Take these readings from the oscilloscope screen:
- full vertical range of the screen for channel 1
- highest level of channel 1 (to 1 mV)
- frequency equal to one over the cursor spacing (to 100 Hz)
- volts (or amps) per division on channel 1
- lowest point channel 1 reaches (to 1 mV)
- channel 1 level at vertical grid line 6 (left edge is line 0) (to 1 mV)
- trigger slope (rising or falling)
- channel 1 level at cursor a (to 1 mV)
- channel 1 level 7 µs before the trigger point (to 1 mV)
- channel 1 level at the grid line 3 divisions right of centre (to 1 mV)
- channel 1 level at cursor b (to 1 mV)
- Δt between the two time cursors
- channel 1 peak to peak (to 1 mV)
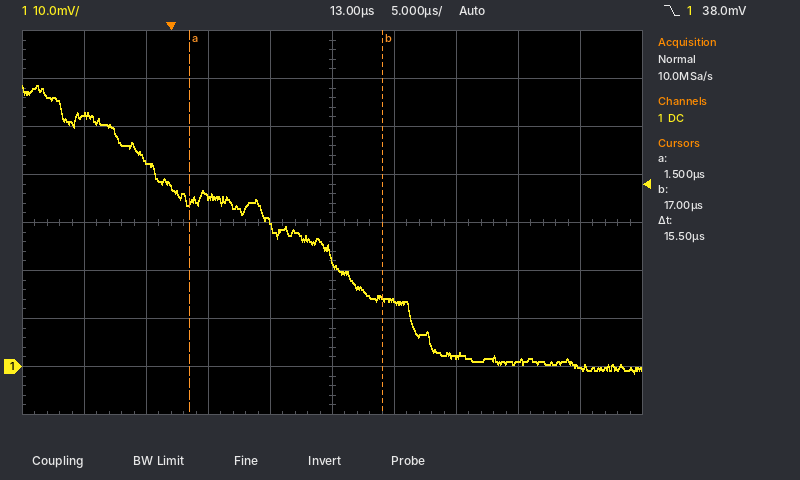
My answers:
80 mV
59 mV
64.5 kHz
10 mV
-1 mV
14 mV
falling
34 mV
52 mV
1 mV
14 mV
15.5 µs
60 mV
